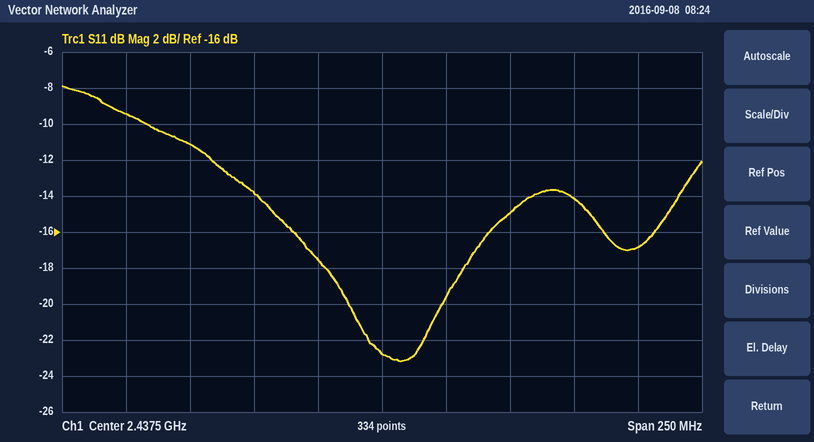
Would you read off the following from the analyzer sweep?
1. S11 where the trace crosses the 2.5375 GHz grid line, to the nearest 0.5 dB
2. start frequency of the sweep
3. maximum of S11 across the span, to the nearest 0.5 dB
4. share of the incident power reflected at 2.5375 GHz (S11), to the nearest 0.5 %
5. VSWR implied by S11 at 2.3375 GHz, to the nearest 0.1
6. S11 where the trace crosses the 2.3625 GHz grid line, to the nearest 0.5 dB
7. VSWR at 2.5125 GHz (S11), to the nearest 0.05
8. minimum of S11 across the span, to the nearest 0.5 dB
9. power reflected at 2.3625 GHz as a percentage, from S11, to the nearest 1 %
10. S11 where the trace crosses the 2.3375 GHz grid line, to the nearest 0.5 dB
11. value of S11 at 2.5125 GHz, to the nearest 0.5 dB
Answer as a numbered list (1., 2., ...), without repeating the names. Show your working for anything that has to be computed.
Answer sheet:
1. -17.0 dB
2. 2.3125 GHz
3. -8.0 dB
4. 10^(-17/10) ≈ 2.0 %
5. |Γ| = 10^(-9.5/20) = 0.3350; VSWR = (1 + 0.3350)/(1 − 0.3350) ≈ 2.0
6. -11.0 dB
7. |Γ| = 10^(-14/20) = 0.1995; VSWR = (1 + 0.1995)/(1 − 0.1995) ≈ 1.50
8. -23.0 dB
9. 10^(-11/10) ≈ 8 %
10. -9.5 dB
11. -14.0 dB
